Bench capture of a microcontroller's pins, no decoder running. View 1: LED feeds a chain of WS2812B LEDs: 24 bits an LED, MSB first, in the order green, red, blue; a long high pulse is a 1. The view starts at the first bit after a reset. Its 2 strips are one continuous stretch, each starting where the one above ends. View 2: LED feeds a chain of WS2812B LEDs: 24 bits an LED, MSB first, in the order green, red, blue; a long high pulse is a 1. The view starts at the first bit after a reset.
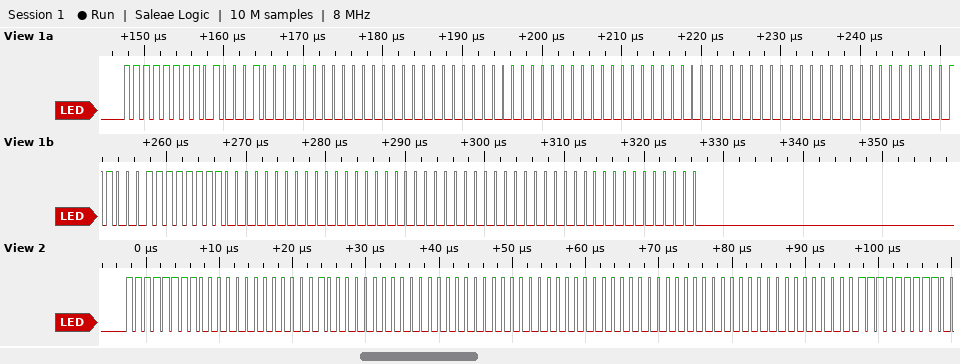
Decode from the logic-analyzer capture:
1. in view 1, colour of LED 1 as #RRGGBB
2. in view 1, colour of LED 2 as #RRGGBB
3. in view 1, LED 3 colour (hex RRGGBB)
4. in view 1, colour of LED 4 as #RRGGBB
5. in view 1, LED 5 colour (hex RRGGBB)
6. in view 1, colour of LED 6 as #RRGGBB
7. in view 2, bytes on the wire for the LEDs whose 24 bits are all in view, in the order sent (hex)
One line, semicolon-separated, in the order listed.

#44FF00; #000000; #000000; #1800FF; #000000; #000000; FF 00 04 00 00 00 00 00 00
